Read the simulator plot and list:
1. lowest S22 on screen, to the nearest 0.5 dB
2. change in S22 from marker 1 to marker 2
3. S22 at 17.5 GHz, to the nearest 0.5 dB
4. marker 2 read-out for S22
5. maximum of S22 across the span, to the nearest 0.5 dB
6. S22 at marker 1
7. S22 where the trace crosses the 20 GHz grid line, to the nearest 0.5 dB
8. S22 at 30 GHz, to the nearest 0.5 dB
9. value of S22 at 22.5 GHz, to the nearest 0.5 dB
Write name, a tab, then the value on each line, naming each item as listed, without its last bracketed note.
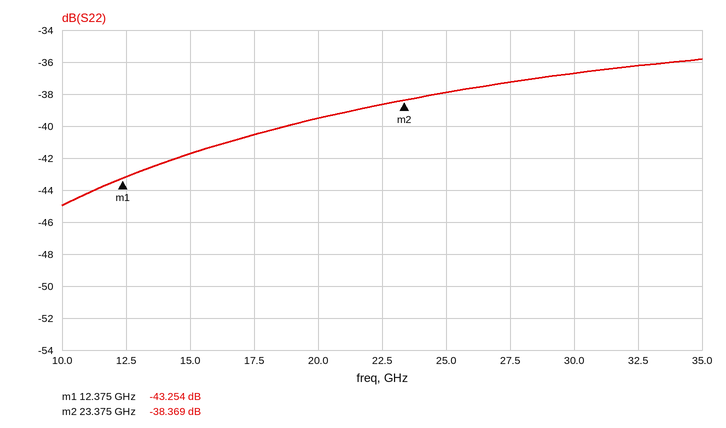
lowest S22 on screen, to the nearest 0.5 dB	-45.0 dB
change in S22 from marker 1 to marker 2	4.885 dB
S22 at 17.5 GHz, to the nearest 0.5 dB	-40.5 dB
marker 2 read-out for S22	-38.369 dB
maximum of S22 across the span, to the nearest 0.5 dB	-36.0 dB
S22 at marker 1	-43.254 dB
S22 where the trace crosses the 20 GHz grid line, to the nearest 0.5 dB	-39.5 dB
S22 at 30 GHz, to the nearest 0.5 dB	-36.5 dB
value of S22 at 22.5 GHz, to the nearest 0.5 dB	-38.5 dB
